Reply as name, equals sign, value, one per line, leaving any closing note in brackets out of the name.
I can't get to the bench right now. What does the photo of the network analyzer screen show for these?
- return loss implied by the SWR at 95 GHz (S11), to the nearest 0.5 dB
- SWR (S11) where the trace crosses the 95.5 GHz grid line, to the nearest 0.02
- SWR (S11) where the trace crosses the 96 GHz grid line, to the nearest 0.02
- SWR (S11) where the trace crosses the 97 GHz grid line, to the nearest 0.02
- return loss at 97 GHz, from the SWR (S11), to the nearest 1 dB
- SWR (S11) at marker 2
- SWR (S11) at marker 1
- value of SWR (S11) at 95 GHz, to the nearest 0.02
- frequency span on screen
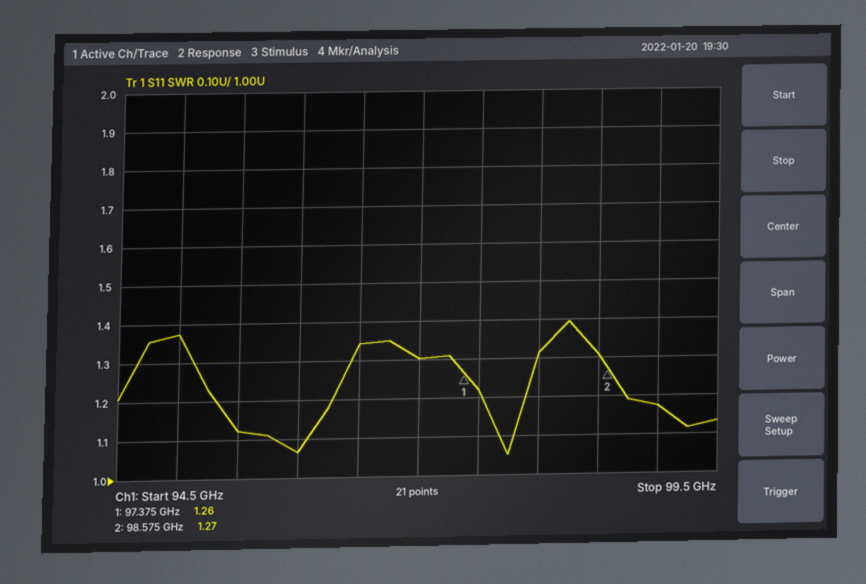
return loss implied by the SWR at 95 GHz (S11), to the nearest 0.5 dB = 16.0 dB
SWR (S11) where the trace crosses the 95.5 GHz grid line, to the nearest 0.02 = 1.12
SWR (S11) where the trace crosses the 96 GHz grid line, to the nearest 0.02 = 1.06
SWR (S11) where the trace crosses the 97 GHz grid line, to the nearest 0.02 = 1.30
return loss at 97 GHz, from the SWR (S11), to the nearest 1 dB = 18 dB
SWR (S11) at marker 2 = 1.27
SWR (S11) at marker 1 = 1.26
value of SWR (S11) at 95 GHz, to the nearest 0.02 = 1.38
frequency span on screen = 5 GHz
